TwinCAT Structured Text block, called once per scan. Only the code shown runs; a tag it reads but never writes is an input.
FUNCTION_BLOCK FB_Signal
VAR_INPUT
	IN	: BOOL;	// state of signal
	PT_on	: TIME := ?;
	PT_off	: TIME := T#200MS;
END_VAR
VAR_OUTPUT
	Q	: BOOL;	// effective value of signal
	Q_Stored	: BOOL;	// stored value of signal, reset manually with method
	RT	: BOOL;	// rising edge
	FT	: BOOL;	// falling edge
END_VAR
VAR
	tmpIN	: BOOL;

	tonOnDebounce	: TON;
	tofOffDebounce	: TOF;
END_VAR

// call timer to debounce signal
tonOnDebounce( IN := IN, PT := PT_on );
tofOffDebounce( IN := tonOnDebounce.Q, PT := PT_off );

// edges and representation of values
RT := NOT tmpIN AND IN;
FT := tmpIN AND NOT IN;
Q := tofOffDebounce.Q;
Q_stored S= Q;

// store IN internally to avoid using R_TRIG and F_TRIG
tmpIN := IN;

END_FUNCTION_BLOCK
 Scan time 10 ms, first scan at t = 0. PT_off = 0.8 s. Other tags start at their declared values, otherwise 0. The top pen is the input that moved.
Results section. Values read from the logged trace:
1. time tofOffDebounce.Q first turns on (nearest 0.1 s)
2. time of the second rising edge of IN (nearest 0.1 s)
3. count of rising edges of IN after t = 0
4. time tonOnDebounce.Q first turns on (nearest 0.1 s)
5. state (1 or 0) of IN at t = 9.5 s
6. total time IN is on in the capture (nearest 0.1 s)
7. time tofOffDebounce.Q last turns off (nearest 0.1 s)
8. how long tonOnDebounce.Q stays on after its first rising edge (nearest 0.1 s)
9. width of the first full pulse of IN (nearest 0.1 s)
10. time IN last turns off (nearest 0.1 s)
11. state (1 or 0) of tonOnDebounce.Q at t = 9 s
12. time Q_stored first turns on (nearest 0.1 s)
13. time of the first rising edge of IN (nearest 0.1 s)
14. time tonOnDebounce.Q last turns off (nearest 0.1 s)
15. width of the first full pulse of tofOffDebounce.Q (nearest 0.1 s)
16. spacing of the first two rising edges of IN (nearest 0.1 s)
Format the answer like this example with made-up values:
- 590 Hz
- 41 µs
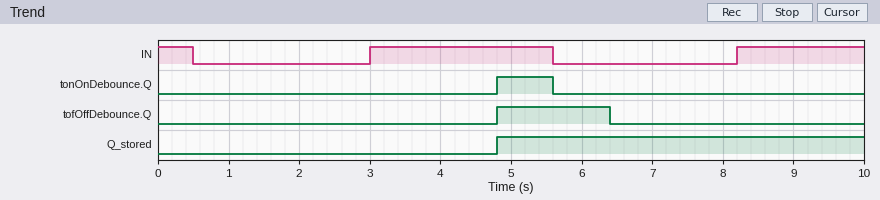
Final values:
- 4.8 s
- 8.2 s
- 2
- 4.8 s
- 1
- 4.9 s
- 6.4 s
- 0.8 s
- 2.6 s
- 5.6 s
- 0
- 4.8 s
- 3.0 s
- 5.6 s
- 1.6 s
- 5.2 s
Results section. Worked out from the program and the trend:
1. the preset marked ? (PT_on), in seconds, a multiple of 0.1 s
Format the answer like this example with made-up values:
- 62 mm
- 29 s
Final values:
- 1.8 s
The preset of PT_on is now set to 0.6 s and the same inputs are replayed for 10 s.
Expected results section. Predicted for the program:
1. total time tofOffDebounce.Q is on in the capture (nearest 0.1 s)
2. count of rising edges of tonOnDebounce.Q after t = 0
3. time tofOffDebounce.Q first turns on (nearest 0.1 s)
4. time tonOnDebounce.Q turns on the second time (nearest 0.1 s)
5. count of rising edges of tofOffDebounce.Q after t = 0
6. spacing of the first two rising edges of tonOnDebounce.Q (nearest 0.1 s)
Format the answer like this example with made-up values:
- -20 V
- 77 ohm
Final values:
- 4.0 s
- 2
- 3.6 s
- 8.8 s
- 2
- 5.2 s
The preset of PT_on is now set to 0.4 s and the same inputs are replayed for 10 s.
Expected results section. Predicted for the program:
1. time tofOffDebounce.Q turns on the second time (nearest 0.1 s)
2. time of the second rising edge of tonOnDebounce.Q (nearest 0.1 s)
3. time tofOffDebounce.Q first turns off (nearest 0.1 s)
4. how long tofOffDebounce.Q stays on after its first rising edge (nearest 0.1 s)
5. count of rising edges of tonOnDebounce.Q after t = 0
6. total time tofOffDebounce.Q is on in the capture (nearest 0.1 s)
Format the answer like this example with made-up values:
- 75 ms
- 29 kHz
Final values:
- 3.4 s
- 3.4 s
- 1.3 s
- 0.9 s
- 3
- 5.3 s
